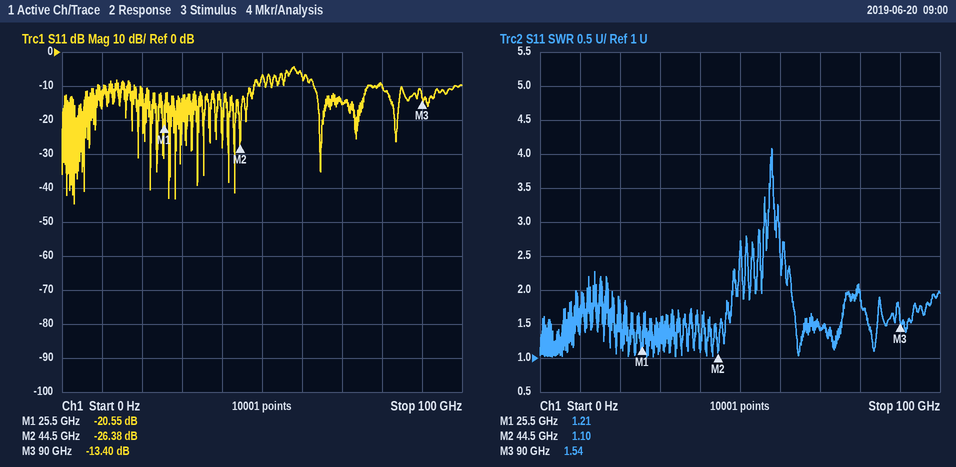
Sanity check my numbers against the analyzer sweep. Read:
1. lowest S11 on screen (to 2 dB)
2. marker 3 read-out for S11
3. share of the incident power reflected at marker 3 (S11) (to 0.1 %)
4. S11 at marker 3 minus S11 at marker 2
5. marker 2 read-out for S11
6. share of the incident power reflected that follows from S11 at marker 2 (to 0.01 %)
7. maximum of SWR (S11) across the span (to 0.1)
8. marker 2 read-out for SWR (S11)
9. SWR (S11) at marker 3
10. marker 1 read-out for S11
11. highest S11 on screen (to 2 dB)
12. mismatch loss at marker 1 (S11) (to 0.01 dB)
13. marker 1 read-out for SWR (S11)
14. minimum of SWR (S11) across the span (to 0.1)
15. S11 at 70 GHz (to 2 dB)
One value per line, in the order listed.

-44 dB
-13.40 dB
4.6 %
12.98 dB
-26.38 dB
0.23 %
4.1
1.10
1.54
-20.55 dB
-4 dB
0.04 dB
1.21
1.0
-16 dB
